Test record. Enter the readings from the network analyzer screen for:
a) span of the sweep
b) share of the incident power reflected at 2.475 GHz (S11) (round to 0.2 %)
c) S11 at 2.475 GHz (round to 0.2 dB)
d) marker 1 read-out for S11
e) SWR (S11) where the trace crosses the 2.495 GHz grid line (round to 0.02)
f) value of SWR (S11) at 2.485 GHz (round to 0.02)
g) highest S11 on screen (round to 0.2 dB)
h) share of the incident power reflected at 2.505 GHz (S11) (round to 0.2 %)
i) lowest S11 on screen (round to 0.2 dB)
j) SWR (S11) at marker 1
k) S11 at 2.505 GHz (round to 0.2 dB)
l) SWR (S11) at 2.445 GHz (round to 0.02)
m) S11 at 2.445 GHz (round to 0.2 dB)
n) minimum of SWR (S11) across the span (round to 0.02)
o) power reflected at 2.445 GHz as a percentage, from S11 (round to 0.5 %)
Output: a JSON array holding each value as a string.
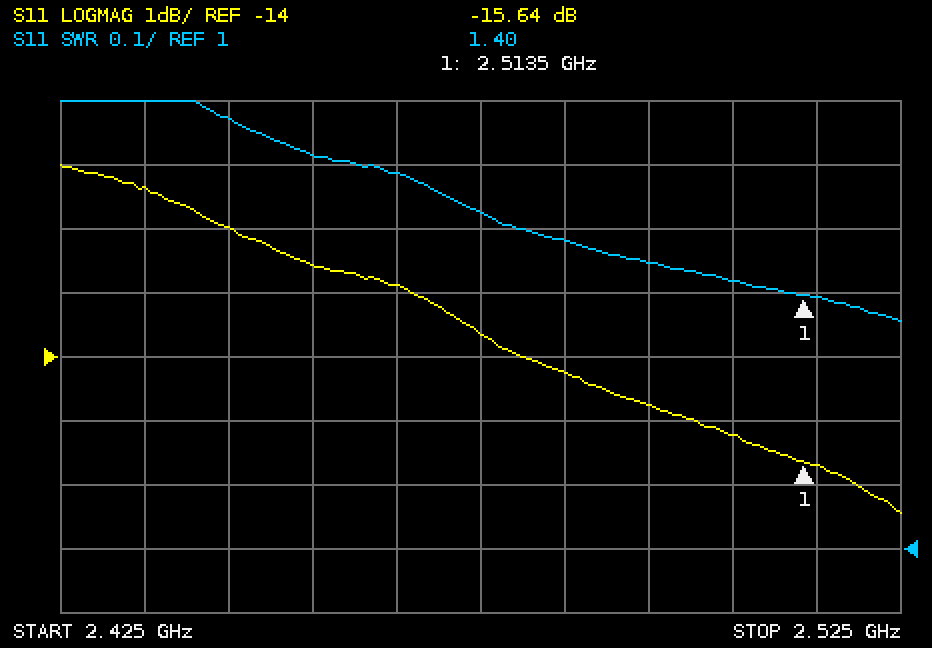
["100 MHz", "4.4 %", "-13.6 dB", "-15.64 dB", "1.44", "1.48", "-11.0 dB", "3.0 %", "-16.4 dB", "1.40", "-15.2 dB", "1.68", "-12.0 dB", "1.36", "6.5 %"]
